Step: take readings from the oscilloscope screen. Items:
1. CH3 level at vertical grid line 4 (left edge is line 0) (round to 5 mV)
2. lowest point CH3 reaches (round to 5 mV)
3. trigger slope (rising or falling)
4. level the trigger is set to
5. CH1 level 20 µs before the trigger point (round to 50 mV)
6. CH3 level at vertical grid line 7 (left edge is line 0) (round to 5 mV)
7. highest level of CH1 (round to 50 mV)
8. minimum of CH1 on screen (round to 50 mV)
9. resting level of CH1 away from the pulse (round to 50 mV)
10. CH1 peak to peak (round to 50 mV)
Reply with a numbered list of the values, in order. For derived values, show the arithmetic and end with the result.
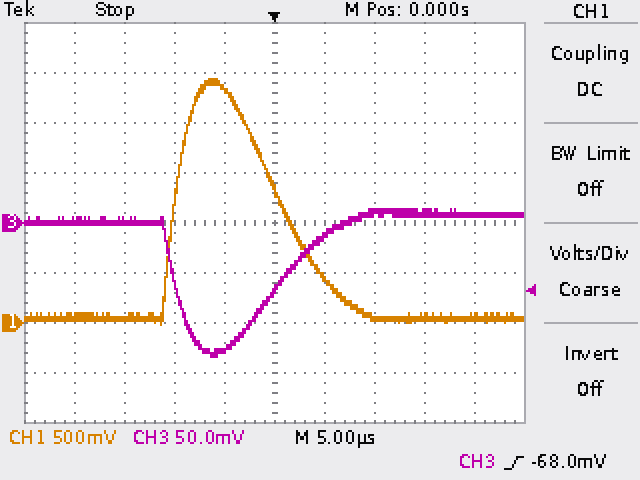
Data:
1. -125 mV
2. -135 mV
3. rising
4. -68.0 mV
5. 50 mV
6. 10 mV
7. 2.45 V
8. 0 mV
9. 50 mV
10. 2.45 V − (0 mV) = 2.45 V
